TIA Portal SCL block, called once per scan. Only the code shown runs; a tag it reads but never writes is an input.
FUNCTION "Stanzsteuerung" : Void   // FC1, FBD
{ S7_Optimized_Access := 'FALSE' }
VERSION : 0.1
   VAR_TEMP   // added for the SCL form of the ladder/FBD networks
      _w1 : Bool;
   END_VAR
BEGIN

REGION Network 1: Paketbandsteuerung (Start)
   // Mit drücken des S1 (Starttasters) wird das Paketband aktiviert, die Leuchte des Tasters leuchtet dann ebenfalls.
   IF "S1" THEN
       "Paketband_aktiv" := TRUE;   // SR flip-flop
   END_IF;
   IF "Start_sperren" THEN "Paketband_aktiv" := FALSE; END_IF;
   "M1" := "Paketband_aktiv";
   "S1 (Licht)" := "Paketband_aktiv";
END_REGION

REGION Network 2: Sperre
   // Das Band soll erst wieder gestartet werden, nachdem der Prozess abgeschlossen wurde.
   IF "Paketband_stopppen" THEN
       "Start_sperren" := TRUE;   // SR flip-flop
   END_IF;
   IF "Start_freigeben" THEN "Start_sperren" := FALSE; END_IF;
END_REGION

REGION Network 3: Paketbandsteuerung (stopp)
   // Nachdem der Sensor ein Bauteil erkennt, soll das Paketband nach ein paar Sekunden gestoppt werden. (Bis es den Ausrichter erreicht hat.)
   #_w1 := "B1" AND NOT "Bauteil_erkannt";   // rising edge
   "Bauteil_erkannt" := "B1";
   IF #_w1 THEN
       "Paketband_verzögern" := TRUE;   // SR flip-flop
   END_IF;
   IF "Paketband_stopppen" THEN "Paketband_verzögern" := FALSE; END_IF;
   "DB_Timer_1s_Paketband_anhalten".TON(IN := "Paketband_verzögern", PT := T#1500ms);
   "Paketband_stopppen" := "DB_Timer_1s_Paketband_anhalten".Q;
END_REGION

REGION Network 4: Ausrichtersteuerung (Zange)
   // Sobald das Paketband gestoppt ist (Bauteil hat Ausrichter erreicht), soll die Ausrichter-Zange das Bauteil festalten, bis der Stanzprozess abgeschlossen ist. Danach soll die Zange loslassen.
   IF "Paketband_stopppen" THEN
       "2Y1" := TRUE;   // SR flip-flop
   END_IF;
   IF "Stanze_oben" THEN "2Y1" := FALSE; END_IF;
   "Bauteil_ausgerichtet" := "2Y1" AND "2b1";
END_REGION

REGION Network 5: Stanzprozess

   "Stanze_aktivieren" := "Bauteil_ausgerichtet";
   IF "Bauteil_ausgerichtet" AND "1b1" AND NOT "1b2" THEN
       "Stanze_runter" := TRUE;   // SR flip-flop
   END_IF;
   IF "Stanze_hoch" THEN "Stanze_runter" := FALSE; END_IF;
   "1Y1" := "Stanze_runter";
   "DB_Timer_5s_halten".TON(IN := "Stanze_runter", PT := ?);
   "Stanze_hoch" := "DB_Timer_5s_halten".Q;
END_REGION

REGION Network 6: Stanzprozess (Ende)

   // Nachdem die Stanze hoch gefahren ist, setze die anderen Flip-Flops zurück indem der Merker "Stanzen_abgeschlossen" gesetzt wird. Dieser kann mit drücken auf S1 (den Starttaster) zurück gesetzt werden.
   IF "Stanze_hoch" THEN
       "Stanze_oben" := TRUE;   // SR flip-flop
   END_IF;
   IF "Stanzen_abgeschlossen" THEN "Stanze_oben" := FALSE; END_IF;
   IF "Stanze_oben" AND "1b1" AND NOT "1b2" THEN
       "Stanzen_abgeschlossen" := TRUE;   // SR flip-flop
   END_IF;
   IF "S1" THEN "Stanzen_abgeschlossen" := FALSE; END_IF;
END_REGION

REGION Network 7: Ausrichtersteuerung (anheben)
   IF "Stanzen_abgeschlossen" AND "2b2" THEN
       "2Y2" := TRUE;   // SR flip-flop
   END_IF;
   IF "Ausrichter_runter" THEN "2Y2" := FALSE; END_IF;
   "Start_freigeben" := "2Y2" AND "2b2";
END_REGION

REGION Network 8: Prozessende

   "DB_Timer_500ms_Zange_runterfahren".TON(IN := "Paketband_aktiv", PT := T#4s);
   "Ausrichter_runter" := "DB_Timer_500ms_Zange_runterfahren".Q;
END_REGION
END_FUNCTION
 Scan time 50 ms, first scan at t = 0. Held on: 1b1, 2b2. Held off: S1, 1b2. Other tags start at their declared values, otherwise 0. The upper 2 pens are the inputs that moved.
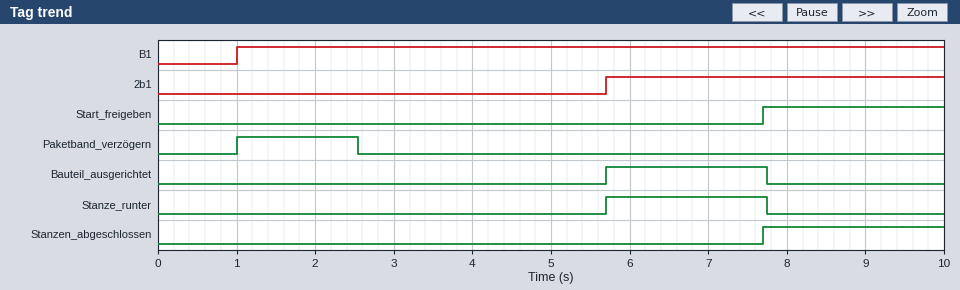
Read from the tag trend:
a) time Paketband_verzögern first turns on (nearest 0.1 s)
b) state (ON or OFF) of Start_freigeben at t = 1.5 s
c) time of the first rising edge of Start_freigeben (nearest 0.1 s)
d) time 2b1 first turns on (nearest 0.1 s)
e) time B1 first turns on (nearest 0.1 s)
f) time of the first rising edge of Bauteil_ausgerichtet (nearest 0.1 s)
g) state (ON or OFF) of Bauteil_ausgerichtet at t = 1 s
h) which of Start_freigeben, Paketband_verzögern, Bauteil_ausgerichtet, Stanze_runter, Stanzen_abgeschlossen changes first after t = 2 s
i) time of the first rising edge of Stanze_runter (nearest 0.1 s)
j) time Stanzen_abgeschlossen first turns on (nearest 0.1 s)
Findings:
1.0 s
OFF
7.7 s
5.7 s
1.0 s
5.7 s
OFF
Paketband_verzögern
5.7 s
7.7 s
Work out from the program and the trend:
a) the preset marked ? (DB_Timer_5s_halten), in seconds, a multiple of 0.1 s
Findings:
2.0 s
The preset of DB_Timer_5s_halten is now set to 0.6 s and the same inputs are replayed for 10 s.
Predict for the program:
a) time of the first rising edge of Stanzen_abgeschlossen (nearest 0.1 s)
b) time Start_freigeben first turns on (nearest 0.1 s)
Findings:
6.3 s
6.3 s
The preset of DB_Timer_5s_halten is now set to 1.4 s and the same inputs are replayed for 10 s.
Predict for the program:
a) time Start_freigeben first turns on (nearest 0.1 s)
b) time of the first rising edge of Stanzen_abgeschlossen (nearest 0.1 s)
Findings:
7.1 s
7.1 s
